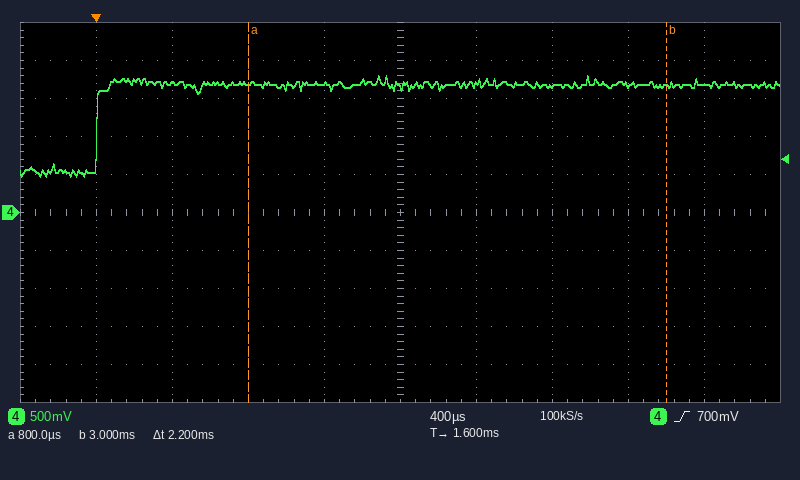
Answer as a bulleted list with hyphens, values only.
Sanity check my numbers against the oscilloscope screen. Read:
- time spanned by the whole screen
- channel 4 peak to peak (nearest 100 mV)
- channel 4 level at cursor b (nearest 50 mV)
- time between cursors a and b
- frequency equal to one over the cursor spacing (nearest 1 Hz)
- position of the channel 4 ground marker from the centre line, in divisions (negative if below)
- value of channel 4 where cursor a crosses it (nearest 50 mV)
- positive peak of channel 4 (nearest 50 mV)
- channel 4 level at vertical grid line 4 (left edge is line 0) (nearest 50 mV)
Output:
- 4 ms
- 1.30 V
- 1.65 V
- 2.2 ms
- 455 Hz
- 0.0 div
- 1.70 V
- 1.80 V
- 1.70 V
